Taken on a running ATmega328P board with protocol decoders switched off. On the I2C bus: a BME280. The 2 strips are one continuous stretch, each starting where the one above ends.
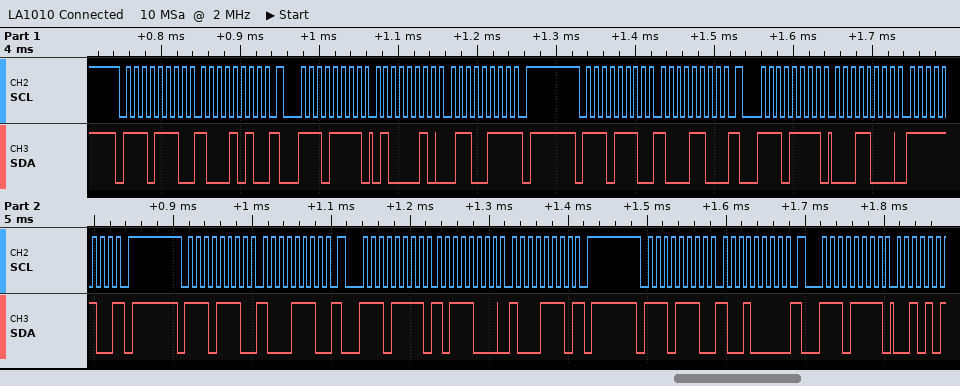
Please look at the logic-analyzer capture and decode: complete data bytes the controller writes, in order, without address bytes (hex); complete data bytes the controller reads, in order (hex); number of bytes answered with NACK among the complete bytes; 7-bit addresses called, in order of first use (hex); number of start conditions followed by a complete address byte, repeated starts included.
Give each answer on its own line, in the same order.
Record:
8A 8C 8E 90
42 67 18 FC B8 8E
3
0x77
8
